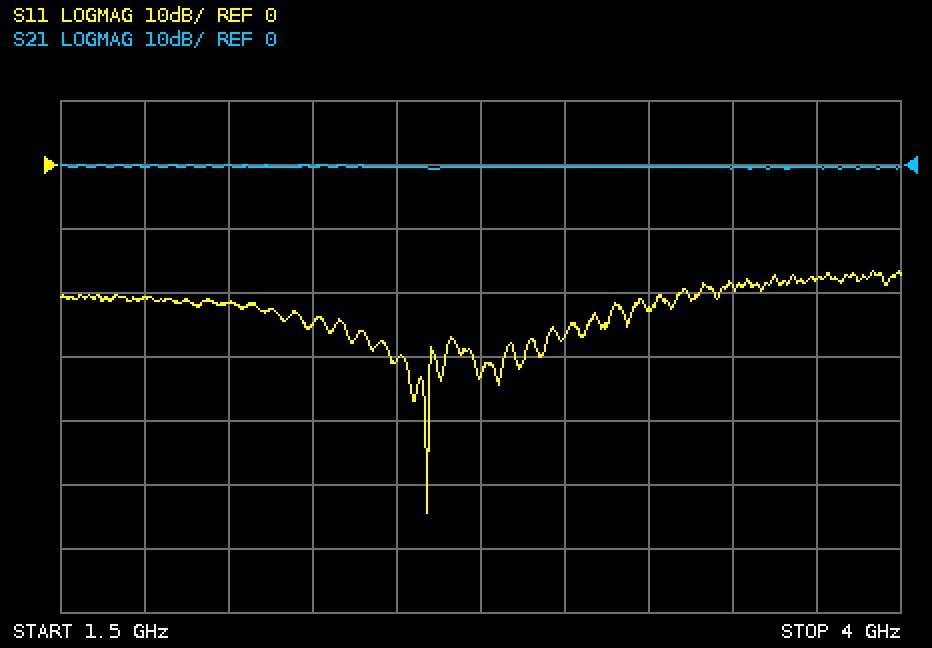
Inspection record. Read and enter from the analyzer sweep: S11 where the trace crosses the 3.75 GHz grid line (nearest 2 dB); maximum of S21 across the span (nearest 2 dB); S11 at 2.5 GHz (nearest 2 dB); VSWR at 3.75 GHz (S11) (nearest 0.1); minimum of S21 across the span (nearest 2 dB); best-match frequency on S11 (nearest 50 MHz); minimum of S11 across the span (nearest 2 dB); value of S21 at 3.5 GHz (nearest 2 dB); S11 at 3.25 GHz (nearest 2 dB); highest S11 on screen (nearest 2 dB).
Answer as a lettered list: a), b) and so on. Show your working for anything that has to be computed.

a) -18 dB
b) 0 dB
c) -30 dB
d) |Γ| = 10^(-18/20) = 0.1259; VSWR = (1 + 0.1259)/(1 − 0.1259) ≈ 1.3
e) 0 dB
f) 2.60 GHz
g) -54 dB
h) 0 dB
i) -22 dB
j) -16 dB
